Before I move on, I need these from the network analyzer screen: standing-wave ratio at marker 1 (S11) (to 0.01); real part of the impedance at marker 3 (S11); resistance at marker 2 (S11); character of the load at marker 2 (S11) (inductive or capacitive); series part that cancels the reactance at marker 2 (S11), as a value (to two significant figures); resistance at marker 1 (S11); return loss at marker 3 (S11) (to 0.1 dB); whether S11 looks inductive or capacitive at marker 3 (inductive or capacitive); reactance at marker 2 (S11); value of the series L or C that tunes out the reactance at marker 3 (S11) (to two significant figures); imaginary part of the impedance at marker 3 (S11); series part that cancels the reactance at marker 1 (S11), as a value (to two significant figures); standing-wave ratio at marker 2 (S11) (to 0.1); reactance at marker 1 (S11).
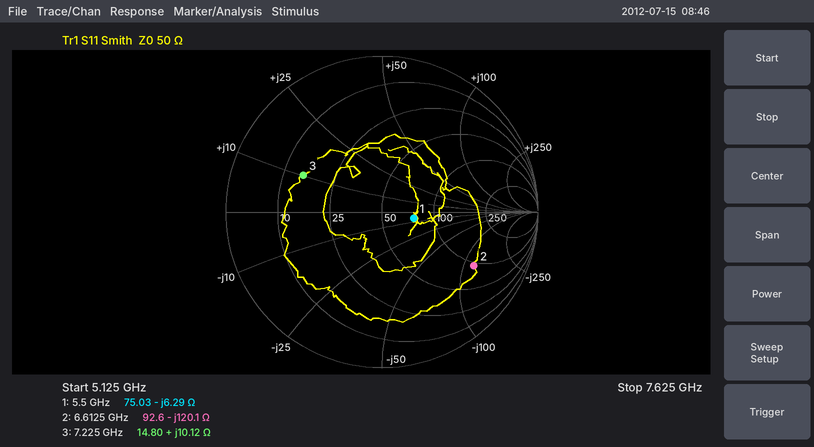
1.52
14.80 Ω
92.6 Ω
capacitive
2.9 nH
75.03 Ω
5.1 dB
inductive
-120.1 Ω
2.2 pF
+10.12 Ω
180 pH
5.3
-6.29 Ω
